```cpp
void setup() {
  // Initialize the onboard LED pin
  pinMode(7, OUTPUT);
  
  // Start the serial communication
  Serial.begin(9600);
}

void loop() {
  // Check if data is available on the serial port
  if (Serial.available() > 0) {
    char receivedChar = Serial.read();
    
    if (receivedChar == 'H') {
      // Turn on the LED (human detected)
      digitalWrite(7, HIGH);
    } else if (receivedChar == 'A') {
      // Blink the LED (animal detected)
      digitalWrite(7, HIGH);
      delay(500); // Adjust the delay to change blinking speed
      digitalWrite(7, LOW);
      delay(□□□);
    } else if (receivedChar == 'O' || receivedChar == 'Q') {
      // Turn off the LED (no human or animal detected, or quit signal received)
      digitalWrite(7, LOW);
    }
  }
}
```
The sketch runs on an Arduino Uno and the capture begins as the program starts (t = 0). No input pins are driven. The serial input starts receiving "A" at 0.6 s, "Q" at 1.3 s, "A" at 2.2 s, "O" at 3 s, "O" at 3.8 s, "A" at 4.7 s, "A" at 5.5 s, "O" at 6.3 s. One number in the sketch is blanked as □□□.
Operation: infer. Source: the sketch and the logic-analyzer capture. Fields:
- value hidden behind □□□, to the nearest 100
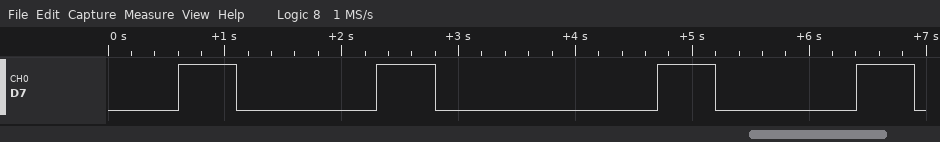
1200
